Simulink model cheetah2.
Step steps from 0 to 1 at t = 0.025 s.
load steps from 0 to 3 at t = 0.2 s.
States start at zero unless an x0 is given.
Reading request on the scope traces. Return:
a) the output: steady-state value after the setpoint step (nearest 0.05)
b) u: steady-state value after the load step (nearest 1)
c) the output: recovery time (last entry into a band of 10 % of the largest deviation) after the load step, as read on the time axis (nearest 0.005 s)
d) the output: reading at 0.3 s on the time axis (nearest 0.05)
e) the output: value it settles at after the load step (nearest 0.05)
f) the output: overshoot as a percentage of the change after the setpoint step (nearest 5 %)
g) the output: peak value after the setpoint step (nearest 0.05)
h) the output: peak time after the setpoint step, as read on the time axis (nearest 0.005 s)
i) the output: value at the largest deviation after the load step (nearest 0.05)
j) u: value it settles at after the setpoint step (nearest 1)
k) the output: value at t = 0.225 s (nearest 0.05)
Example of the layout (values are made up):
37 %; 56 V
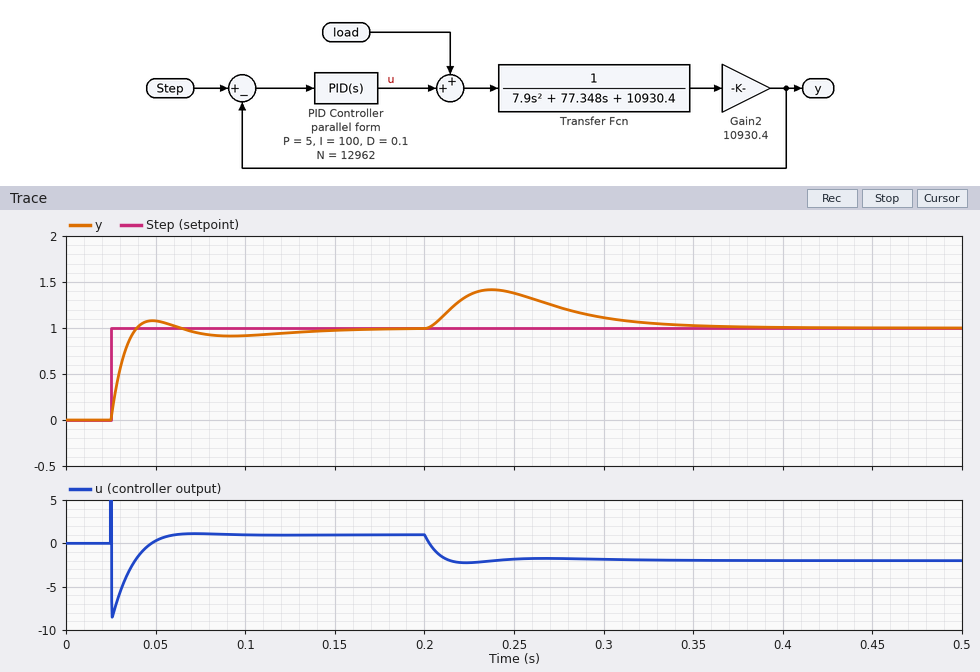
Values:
1.00; -2; 0.335 s; 1.10; 1.00; 10 %; 1.10; 0.050 s; 1.40; 1; 1.35
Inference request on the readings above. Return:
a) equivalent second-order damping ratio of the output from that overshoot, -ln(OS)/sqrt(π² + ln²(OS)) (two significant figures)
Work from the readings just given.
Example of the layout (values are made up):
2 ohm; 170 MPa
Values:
0.59
